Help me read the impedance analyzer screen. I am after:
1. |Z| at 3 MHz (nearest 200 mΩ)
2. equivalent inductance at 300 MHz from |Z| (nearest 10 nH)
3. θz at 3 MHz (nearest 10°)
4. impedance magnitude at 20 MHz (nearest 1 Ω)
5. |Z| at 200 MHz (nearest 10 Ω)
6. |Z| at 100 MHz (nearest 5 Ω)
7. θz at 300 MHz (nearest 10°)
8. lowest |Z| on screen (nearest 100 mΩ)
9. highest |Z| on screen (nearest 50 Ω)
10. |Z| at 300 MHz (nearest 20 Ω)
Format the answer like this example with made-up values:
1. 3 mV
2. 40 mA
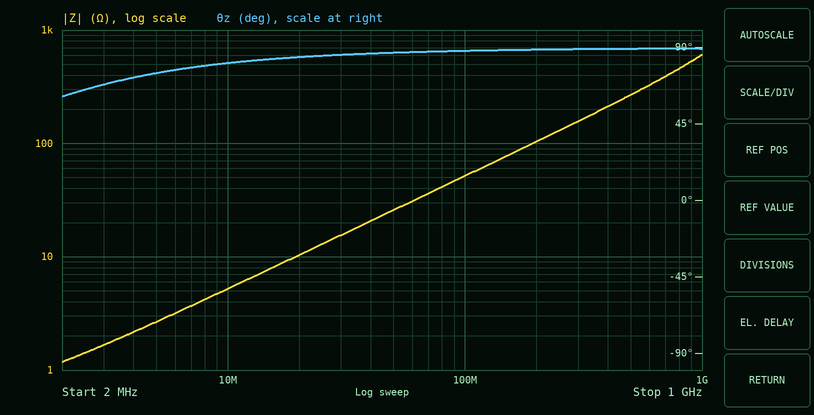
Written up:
1. 1.6 Ω
2. 80 nH
3. 70°
4. 10 Ω
5. 100 Ω
6. 50 Ω
7. 90°
8. 1.2 Ω
9. 600 Ω
10. 160 Ω
